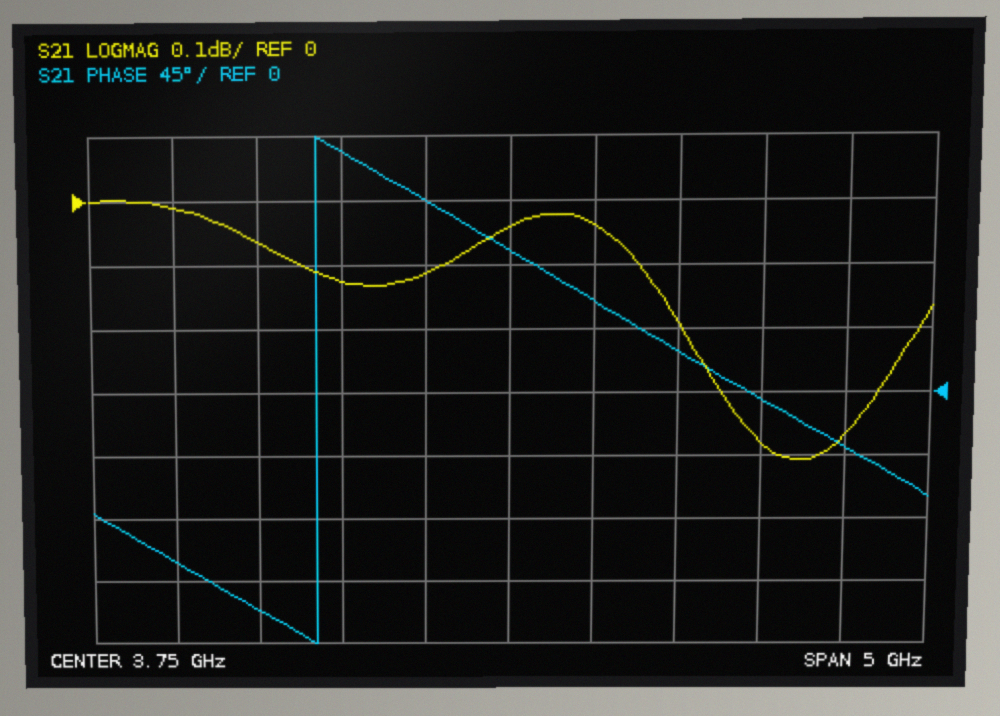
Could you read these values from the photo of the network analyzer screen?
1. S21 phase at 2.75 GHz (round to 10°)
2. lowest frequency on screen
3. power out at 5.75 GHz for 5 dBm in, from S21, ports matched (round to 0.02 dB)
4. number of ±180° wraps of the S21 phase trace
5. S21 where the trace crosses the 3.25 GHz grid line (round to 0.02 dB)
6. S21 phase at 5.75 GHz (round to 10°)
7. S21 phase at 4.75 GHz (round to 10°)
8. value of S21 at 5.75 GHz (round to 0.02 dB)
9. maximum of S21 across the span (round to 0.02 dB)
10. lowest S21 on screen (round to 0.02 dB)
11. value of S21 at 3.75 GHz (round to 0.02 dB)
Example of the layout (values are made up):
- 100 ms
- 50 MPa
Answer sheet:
- 170°
- 1.25 GHz
- 4.64 dBm
- 1
- -0.12 dB
- -40°
- 30°
- -0.36 dB
- 0.00 dB
- -0.40 dB
- -0.04 dB
